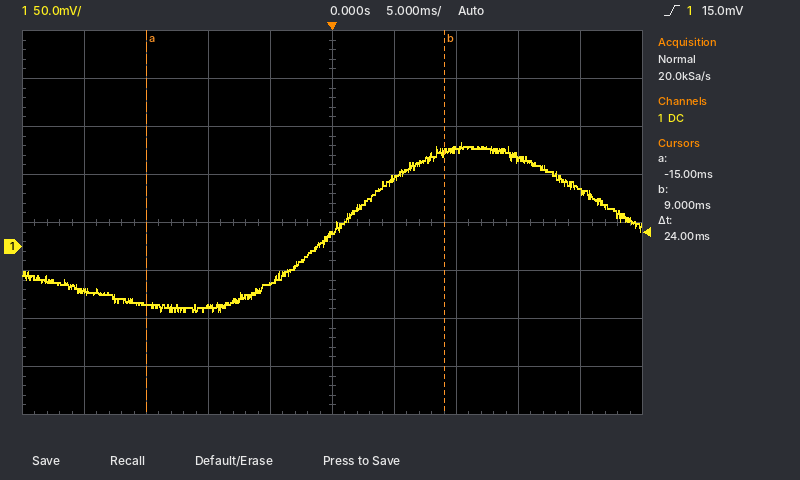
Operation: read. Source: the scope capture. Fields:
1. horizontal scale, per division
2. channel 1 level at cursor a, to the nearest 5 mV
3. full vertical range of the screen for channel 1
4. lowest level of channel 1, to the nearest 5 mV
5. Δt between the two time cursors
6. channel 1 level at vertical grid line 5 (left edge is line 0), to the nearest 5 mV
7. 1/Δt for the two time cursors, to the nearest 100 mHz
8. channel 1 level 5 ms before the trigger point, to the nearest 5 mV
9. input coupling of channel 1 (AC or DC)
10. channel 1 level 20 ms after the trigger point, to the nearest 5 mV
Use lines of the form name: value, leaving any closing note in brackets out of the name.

horizontal scale, per division: 5 ms
channel 1 level at cursor a, to the nearest 5 mV: -60 mV
full vertical range of the screen for channel 1: 400 mV
lowest level of channel 1, to the nearest 5 mV: -70 mV
Δt between the two time cursors: 24 ms
channel 1 level at vertical grid line 5 (left edge is line 0), to the nearest 5 mV: 15 mV
1/Δt for the two time cursors, to the nearest 100 mHz: 41.7 Hz
channel 1 level 5 ms before the trigger point, to the nearest 5 mV: -40 mV
input coupling of channel 1: DC
channel 1 level 20 ms after the trigger point, to the nearest 5 mV: 60 mV
